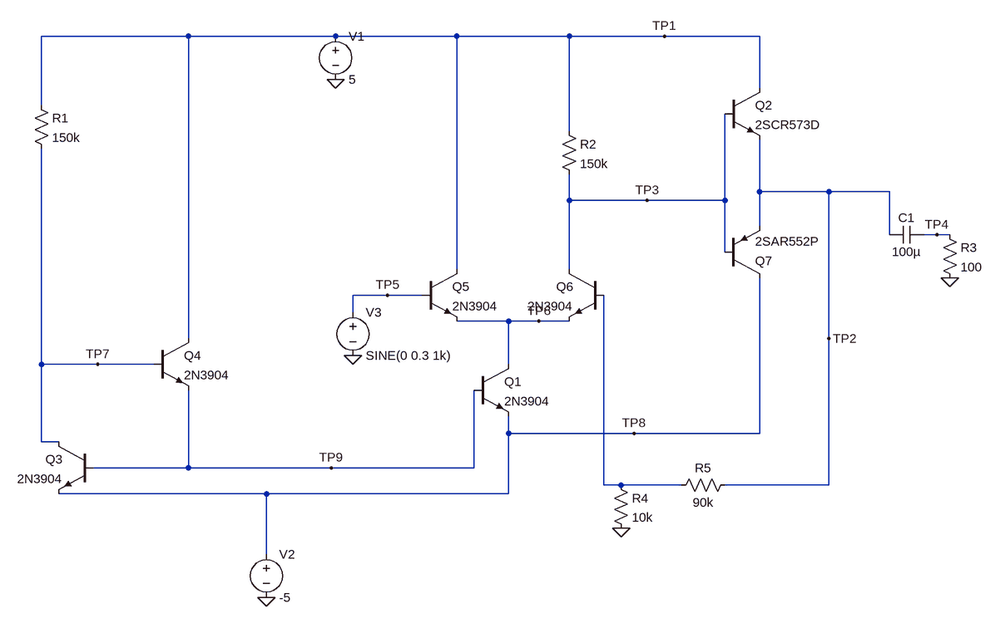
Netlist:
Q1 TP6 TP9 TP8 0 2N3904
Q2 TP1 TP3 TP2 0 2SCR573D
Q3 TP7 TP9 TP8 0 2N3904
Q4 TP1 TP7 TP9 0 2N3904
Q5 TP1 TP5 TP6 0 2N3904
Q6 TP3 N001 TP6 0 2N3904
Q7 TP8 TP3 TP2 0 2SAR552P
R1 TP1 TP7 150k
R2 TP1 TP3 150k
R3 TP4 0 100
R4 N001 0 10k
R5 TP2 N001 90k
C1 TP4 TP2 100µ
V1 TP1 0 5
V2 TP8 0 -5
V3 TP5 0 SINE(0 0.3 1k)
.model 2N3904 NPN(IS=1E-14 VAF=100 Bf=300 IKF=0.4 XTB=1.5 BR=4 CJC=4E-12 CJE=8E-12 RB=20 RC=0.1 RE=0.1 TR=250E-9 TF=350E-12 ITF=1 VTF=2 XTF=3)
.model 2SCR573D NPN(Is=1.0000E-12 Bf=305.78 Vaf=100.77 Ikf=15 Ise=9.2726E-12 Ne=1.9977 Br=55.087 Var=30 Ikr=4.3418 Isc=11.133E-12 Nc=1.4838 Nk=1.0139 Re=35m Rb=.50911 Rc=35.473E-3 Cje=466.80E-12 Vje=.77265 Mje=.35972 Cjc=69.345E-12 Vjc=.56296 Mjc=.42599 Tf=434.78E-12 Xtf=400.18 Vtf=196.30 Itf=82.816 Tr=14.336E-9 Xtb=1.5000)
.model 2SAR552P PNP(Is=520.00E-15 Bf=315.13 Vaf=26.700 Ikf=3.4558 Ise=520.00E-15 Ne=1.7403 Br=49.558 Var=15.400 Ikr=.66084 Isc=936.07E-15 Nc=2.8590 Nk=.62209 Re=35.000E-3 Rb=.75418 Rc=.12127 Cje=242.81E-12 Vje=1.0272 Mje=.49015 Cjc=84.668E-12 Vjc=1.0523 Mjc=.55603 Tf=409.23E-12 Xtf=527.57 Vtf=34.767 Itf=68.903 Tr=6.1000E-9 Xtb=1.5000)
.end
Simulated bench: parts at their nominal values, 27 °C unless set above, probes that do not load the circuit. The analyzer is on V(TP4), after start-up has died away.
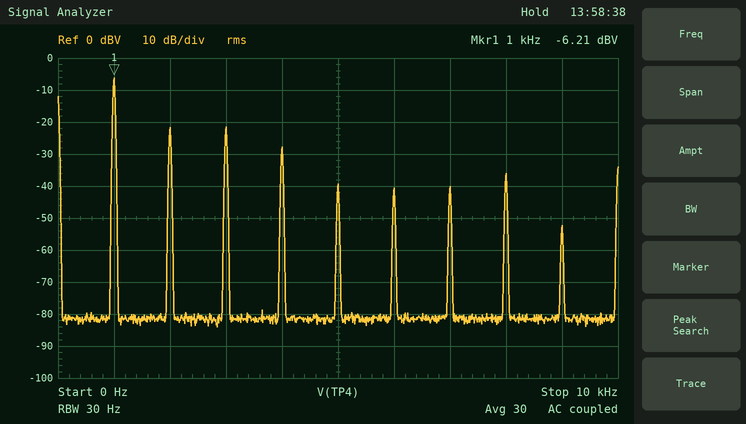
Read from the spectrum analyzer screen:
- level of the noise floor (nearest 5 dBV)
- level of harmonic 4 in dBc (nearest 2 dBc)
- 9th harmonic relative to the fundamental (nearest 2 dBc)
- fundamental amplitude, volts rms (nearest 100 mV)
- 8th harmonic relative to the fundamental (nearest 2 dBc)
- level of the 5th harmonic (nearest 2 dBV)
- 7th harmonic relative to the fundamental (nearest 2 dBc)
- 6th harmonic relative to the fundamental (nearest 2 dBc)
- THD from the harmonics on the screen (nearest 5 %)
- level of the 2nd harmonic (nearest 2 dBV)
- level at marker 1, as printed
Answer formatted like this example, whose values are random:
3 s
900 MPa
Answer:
-80 dBV
-22 dBc
-46 dBc
500 mV
-30 dBc
-40 dBV
-34 dBc
-34 dBc
25 %
-22 dBV
-6.21 dBV
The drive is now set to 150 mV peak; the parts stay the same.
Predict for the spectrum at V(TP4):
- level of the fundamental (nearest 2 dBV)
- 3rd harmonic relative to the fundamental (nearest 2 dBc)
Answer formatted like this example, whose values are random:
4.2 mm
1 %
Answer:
-10 dBV
-28 dBc
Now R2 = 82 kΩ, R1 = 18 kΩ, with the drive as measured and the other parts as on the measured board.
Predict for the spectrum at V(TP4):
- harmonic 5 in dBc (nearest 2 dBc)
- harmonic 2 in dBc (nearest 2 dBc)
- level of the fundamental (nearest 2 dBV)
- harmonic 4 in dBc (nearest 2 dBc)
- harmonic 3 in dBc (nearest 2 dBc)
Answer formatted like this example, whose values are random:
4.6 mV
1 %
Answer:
-26 dBc
-10 dBc
-4 dBV
-20 dBc
-34 dBc
